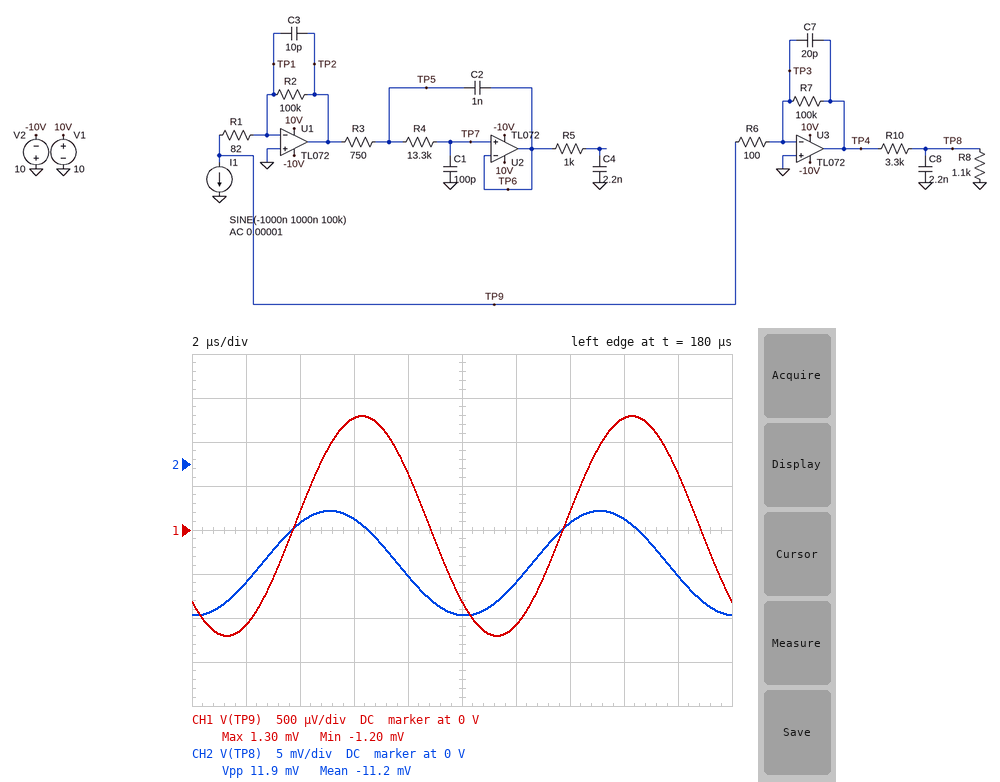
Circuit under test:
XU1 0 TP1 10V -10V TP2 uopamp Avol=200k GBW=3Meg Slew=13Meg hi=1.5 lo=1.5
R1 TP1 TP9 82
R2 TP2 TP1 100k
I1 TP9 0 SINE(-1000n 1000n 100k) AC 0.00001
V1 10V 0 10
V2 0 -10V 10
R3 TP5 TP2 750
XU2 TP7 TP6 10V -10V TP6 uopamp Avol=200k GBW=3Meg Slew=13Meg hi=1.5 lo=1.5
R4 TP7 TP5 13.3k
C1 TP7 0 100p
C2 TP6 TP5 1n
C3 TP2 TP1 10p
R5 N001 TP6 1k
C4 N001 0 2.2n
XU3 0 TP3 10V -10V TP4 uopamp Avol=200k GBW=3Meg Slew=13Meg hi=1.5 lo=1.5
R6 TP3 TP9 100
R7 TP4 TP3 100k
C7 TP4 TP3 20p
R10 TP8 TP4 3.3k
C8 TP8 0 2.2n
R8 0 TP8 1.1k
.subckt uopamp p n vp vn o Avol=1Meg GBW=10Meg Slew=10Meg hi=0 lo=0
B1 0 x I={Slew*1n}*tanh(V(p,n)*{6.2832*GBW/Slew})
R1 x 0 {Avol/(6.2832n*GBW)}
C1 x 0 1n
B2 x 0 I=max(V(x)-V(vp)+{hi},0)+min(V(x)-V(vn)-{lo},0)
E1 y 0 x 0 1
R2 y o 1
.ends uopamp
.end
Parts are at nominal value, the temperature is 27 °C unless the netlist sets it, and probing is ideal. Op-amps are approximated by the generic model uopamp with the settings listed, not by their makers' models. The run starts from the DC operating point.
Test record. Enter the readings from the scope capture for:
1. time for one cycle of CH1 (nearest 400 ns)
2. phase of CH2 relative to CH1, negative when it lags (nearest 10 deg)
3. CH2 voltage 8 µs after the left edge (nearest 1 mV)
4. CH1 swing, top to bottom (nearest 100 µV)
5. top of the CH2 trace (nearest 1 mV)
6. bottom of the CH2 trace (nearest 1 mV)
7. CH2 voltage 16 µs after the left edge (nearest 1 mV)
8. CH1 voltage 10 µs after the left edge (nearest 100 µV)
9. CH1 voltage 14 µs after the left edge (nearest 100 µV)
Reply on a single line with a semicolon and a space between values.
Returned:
10.0 µs; 40 deg; -13 mV; 2.5 mV; -5 mV; -17 mV; -6 mV; -800 µV; 200 µV
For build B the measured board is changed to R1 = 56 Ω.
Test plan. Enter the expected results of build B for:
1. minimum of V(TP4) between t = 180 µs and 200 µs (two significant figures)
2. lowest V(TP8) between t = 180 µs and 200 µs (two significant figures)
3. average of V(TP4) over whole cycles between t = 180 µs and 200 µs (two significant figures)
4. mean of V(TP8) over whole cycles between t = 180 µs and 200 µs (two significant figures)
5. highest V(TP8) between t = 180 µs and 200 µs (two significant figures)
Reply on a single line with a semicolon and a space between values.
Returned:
-72 mV; -15 mV; -36 mV; -9.0 mV; -3.1 mV
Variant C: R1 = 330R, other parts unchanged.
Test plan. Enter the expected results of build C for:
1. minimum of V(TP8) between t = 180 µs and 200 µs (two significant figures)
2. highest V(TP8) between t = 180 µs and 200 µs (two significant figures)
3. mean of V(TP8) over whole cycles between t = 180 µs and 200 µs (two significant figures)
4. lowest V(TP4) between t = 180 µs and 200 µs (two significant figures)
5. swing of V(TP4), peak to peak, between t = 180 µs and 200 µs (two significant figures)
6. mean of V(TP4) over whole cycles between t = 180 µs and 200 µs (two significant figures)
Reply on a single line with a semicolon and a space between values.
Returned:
-25 mV; -13 mV; -19 mV; -110 mV; 73 mV; -77 mV
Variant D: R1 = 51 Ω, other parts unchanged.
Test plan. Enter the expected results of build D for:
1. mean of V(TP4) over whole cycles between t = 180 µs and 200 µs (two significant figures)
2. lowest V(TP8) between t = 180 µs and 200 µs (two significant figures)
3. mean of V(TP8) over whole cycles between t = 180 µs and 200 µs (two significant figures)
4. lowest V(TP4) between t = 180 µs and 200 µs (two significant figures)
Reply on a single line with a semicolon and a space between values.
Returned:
-34 mV; -14 mV; -8.5 mV; -70 mV
